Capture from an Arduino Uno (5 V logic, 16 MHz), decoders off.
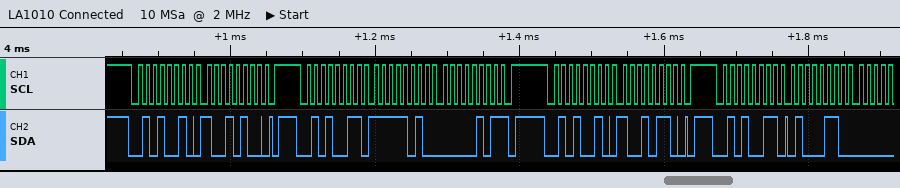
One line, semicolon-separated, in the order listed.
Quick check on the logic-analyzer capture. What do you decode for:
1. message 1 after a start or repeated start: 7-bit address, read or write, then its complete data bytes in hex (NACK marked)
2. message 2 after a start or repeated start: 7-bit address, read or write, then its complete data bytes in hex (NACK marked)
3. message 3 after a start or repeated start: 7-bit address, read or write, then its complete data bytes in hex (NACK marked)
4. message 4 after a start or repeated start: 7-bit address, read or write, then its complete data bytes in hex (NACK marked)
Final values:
0x29 write: 94; 0x29 read: FA 05 NACK; 0x29 write: 96; 0x29 read: 46
